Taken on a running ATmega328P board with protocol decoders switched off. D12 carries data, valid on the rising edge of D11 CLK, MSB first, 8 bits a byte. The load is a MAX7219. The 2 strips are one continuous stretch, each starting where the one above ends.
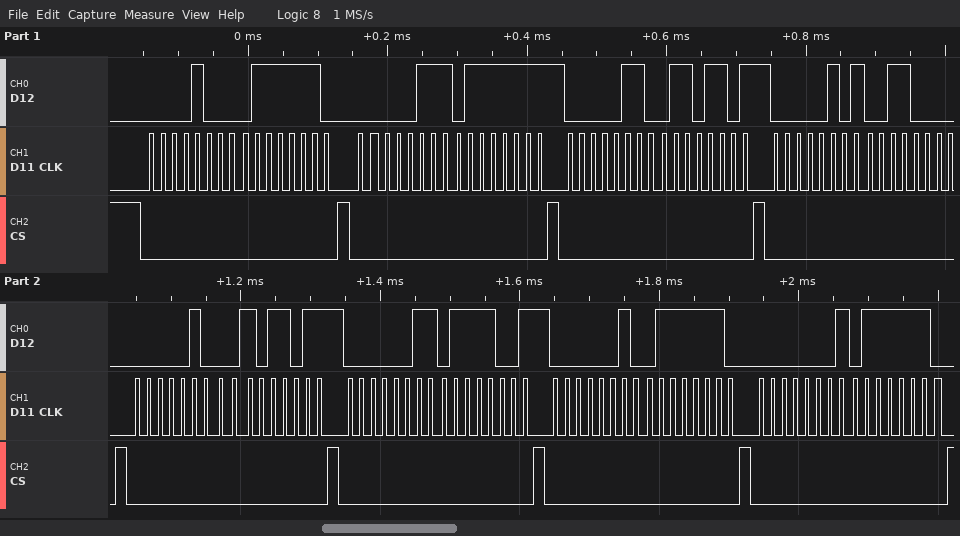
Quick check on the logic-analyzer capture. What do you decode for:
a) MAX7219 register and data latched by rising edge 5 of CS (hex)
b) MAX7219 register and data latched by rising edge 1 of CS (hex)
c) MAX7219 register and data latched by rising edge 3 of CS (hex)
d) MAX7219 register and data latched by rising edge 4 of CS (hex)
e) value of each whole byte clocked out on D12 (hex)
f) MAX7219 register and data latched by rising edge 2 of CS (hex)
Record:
register 0x4, data 0x5B
register 0x8, data 0x7E
register 0x6, data 0x6D
register 0x5, data 0x30
08 7E 07 7F 06 6D 05 30 04 5B 03 79 02 7E 01 7E
register 0x7, data 0x7F
